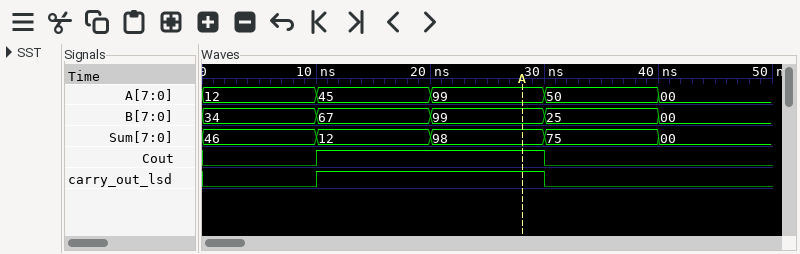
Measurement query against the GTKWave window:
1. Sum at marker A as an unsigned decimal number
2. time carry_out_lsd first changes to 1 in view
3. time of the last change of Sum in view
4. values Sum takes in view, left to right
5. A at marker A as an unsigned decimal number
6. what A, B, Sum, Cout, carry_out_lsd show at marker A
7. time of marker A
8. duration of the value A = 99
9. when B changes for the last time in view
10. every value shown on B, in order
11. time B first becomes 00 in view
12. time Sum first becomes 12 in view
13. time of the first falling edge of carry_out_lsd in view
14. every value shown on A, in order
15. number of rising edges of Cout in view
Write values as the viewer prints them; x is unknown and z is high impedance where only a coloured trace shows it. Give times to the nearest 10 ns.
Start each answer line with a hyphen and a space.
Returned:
- 152
- 10 ns
- 40 ns
- 46, 12, 98, 75, 00
- 153
- A=99, B=99, Sum=98, Cout=1, carry_out_lsd=1
- 30 ns
- 10 ns
- 40 ns
- 34, 67, 99, 25, 00
- 40 ns
- 10 ns
- 30 ns
- 12, 45, 99, 50, 00
- 1
